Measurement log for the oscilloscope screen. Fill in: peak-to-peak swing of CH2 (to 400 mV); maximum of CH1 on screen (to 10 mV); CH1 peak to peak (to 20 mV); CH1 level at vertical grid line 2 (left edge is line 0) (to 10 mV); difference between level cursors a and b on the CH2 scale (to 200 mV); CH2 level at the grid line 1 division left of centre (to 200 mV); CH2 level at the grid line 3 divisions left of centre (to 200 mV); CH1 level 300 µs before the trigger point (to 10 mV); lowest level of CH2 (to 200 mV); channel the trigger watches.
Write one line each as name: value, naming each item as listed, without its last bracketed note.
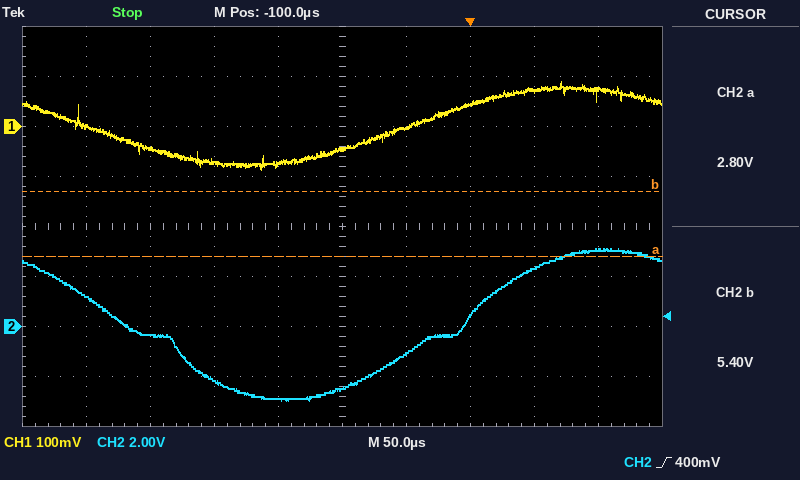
peak-to-peak swing of CH2: 6.0 V
maximum of CH1 on screen: 90 mV
CH1 peak to peak: 180 mV
CH1 level at vertical grid line 2 (left edge is line 0): -40 mV
difference between level cursors a and b on the CH2 scale: 2.6 V
CH2 level at the grid line 1 division left of centre: -2.8 V
CH2 level at the grid line 3 divisions left of centre: -400 mV
CH1 level 300 µs before the trigger point: 0 mV
lowest level of CH2: -3.0 V
channel the trigger watches: CH2
